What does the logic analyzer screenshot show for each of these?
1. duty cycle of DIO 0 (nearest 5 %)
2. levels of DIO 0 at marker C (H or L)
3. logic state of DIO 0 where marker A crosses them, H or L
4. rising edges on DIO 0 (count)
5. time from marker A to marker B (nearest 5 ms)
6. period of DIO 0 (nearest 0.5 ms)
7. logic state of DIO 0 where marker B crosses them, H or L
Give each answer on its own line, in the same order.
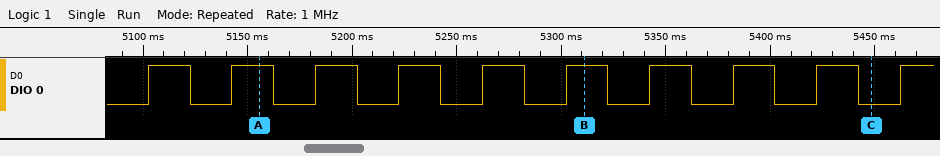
50 %
DIO 0=L
DIO 0=H
10
155 ms
40 ms
DIO 0=H
